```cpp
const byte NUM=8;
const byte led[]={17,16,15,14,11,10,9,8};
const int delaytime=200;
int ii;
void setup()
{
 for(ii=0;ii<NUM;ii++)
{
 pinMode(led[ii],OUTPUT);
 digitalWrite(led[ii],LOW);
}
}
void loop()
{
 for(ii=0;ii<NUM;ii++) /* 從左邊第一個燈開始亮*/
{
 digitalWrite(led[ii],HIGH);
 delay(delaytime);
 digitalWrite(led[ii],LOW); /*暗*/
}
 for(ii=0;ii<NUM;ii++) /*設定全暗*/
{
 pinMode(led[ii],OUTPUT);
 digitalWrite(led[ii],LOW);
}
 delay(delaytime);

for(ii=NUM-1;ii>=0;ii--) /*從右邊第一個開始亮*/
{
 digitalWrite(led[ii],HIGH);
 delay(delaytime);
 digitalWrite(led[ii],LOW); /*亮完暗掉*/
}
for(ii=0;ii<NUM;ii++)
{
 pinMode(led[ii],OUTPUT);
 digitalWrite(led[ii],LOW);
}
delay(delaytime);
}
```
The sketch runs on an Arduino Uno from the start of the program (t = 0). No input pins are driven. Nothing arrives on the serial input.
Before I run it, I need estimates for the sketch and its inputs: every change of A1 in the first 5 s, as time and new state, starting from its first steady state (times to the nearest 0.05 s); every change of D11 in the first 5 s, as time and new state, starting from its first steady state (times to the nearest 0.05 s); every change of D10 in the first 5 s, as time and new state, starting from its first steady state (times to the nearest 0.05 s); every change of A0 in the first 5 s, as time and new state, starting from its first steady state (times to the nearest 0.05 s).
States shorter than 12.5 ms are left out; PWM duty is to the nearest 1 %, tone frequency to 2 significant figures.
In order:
0 s low; 0.4 s high; 0.6 s low; 2.8 s high; 3 s low; 4 s high; 4.2 s low
0 s low; 0.8 s high; 1 s low; 2.4 s high; 2.6 s low; 4.4 s high; 4.6 s low
0 s low; 1 s high; 1.2 s low; 2.2 s high; 2.4 s low; 4.6 s high; 4.8 s low
0 s low; 0.6 s high; 0.8 s low; 2.6 s high; 2.8 s low; 4.2 s high; 4.4 s low
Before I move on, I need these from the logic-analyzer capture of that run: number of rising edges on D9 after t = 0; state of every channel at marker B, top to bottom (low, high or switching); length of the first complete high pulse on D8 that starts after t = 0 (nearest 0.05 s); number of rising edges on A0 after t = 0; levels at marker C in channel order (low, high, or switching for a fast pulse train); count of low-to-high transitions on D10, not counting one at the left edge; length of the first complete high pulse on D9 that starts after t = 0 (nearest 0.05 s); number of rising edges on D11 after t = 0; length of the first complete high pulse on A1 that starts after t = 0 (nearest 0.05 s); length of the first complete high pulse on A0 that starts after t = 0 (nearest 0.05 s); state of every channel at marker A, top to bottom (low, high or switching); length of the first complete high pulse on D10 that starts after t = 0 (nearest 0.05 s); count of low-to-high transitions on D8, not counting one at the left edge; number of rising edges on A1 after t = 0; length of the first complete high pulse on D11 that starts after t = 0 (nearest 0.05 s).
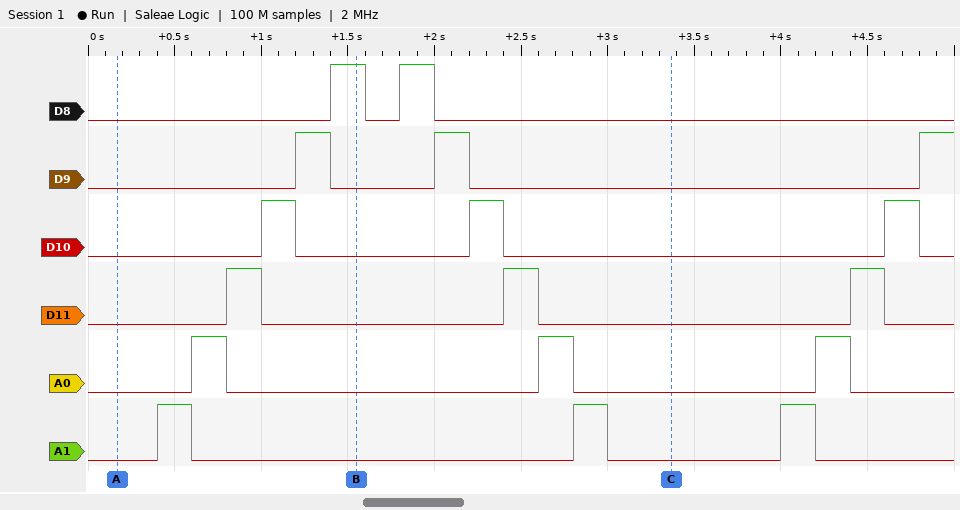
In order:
3
D8 high, D9 low, D10 low, D11 low, A0 low, A1 low
0.20 s
3
D8 low, D9 low, D10 low, D11 low, A0 low, A1 low
3
0.20 s
3
0.20 s
0.20 s
D8 low, D9 low, D10 low, D11 low, A0 low, A1 low
0.20 s
2
3
0.20 s
